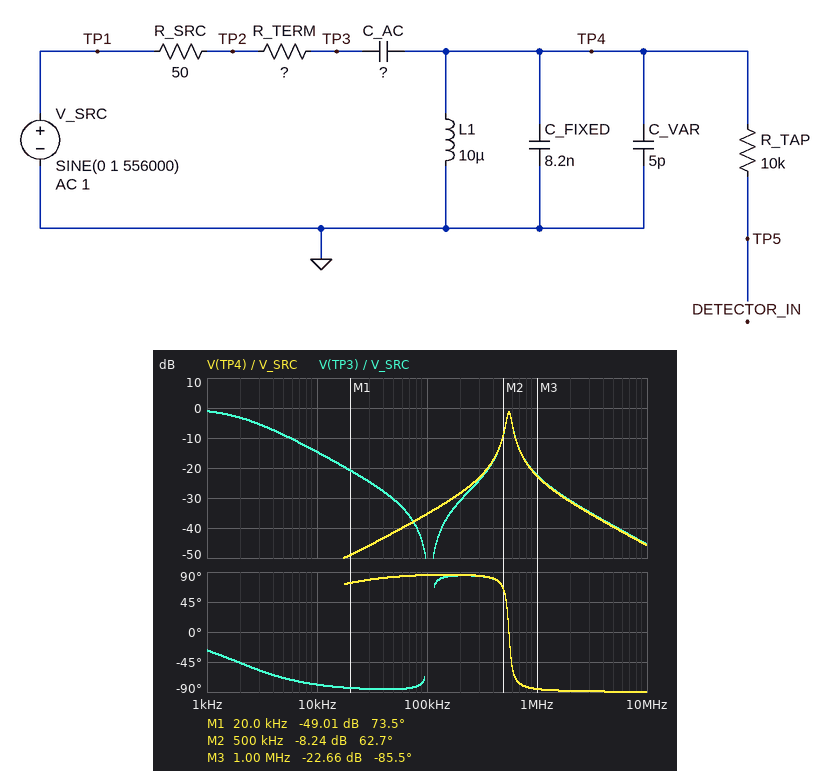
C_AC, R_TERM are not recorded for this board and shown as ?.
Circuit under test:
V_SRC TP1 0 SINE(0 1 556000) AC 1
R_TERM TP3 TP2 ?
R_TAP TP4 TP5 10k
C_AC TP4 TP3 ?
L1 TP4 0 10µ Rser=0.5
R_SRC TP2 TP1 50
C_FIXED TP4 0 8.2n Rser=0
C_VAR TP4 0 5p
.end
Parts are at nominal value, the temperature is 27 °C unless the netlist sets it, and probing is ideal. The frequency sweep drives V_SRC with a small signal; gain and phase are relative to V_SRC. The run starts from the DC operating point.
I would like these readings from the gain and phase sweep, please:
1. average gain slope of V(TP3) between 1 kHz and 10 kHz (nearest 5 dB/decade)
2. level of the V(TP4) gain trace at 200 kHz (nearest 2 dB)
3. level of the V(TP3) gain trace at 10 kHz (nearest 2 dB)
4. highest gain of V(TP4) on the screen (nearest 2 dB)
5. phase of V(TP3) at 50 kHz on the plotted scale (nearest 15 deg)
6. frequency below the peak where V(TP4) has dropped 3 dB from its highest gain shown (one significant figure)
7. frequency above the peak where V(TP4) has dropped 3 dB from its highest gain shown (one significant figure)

-15 dB/decade
-28 dB
-14 dB
-2 dB
-90 deg
500 kHz
600 kHz
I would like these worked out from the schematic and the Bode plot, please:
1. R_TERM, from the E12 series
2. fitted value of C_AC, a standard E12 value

330 Ω
220 nF
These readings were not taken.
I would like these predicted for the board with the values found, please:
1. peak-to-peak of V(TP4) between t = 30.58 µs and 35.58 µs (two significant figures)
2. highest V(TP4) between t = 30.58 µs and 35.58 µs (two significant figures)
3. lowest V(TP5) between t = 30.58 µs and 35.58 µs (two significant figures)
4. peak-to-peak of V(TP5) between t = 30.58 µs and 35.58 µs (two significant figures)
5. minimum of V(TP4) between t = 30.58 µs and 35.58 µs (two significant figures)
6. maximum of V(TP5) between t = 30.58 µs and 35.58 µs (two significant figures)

1.7 V
860 mV
-860 mV
1.7 V
-860 mV
860 mV
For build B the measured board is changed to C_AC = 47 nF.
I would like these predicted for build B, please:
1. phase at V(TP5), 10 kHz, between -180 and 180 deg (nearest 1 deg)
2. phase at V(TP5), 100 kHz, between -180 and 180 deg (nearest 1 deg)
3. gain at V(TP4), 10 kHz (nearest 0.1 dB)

93 deg
89 deg
-56.0 dB
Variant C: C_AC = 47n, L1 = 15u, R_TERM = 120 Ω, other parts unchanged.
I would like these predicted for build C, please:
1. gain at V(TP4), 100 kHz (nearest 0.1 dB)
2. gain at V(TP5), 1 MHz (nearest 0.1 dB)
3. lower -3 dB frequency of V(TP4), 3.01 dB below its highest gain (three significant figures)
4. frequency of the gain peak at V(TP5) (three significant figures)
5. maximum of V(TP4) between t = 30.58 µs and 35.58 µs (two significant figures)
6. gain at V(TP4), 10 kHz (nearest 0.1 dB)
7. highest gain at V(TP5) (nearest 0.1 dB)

-24.8 dB
-17.0 dB
396 kHz
452 kHz
510 mV
-51.0 dB
-0.4 dB
